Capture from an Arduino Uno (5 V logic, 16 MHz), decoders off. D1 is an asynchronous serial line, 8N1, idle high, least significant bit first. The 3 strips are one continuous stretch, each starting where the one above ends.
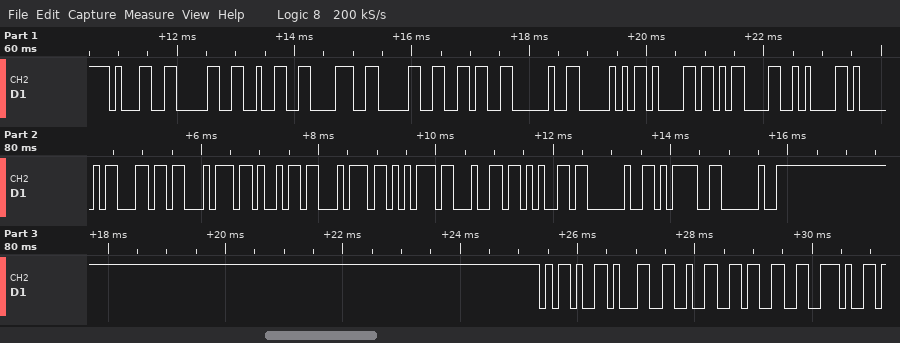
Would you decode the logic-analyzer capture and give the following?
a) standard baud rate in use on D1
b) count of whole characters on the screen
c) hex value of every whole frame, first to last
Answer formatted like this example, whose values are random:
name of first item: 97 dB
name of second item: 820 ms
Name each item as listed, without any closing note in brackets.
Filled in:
standard baud rate in use on D1: 9600 baud
count of whole characters on the screen: 27
hex value of every whole frame, first to last: 31 30 32 38 30 36 20 50 61 0D 0A 41 6C 74 69 74 75 64 65 20 3D 20 2D 31 32 33 2E
